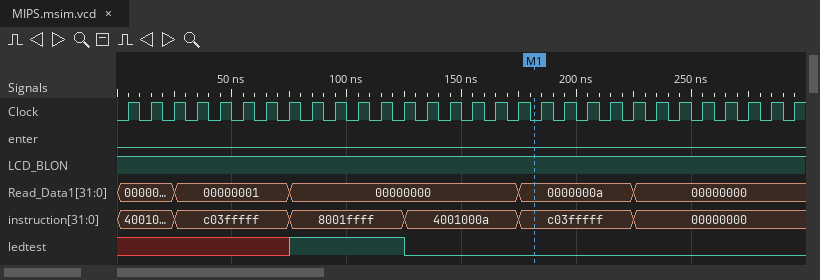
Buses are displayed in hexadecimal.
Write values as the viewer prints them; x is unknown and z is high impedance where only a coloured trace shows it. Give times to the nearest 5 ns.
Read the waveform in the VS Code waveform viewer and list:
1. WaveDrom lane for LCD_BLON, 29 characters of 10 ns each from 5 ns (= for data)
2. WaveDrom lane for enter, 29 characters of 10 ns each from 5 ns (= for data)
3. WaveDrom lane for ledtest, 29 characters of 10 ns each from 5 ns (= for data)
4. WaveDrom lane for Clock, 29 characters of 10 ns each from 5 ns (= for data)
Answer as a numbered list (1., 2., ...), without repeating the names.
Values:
1. {name: 'LCD_BLON', wave: '1............................'}
2. {name: 'enter', wave: '0............................'}
3. {name: 'ledtest', wave: 'x......1....0................'}
4. {name: 'Clock', wave: 'p............................'}
